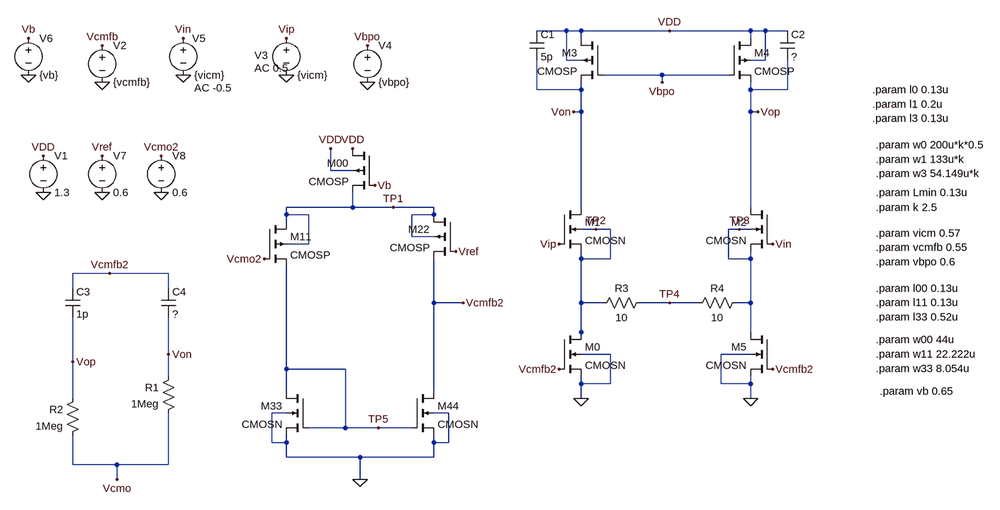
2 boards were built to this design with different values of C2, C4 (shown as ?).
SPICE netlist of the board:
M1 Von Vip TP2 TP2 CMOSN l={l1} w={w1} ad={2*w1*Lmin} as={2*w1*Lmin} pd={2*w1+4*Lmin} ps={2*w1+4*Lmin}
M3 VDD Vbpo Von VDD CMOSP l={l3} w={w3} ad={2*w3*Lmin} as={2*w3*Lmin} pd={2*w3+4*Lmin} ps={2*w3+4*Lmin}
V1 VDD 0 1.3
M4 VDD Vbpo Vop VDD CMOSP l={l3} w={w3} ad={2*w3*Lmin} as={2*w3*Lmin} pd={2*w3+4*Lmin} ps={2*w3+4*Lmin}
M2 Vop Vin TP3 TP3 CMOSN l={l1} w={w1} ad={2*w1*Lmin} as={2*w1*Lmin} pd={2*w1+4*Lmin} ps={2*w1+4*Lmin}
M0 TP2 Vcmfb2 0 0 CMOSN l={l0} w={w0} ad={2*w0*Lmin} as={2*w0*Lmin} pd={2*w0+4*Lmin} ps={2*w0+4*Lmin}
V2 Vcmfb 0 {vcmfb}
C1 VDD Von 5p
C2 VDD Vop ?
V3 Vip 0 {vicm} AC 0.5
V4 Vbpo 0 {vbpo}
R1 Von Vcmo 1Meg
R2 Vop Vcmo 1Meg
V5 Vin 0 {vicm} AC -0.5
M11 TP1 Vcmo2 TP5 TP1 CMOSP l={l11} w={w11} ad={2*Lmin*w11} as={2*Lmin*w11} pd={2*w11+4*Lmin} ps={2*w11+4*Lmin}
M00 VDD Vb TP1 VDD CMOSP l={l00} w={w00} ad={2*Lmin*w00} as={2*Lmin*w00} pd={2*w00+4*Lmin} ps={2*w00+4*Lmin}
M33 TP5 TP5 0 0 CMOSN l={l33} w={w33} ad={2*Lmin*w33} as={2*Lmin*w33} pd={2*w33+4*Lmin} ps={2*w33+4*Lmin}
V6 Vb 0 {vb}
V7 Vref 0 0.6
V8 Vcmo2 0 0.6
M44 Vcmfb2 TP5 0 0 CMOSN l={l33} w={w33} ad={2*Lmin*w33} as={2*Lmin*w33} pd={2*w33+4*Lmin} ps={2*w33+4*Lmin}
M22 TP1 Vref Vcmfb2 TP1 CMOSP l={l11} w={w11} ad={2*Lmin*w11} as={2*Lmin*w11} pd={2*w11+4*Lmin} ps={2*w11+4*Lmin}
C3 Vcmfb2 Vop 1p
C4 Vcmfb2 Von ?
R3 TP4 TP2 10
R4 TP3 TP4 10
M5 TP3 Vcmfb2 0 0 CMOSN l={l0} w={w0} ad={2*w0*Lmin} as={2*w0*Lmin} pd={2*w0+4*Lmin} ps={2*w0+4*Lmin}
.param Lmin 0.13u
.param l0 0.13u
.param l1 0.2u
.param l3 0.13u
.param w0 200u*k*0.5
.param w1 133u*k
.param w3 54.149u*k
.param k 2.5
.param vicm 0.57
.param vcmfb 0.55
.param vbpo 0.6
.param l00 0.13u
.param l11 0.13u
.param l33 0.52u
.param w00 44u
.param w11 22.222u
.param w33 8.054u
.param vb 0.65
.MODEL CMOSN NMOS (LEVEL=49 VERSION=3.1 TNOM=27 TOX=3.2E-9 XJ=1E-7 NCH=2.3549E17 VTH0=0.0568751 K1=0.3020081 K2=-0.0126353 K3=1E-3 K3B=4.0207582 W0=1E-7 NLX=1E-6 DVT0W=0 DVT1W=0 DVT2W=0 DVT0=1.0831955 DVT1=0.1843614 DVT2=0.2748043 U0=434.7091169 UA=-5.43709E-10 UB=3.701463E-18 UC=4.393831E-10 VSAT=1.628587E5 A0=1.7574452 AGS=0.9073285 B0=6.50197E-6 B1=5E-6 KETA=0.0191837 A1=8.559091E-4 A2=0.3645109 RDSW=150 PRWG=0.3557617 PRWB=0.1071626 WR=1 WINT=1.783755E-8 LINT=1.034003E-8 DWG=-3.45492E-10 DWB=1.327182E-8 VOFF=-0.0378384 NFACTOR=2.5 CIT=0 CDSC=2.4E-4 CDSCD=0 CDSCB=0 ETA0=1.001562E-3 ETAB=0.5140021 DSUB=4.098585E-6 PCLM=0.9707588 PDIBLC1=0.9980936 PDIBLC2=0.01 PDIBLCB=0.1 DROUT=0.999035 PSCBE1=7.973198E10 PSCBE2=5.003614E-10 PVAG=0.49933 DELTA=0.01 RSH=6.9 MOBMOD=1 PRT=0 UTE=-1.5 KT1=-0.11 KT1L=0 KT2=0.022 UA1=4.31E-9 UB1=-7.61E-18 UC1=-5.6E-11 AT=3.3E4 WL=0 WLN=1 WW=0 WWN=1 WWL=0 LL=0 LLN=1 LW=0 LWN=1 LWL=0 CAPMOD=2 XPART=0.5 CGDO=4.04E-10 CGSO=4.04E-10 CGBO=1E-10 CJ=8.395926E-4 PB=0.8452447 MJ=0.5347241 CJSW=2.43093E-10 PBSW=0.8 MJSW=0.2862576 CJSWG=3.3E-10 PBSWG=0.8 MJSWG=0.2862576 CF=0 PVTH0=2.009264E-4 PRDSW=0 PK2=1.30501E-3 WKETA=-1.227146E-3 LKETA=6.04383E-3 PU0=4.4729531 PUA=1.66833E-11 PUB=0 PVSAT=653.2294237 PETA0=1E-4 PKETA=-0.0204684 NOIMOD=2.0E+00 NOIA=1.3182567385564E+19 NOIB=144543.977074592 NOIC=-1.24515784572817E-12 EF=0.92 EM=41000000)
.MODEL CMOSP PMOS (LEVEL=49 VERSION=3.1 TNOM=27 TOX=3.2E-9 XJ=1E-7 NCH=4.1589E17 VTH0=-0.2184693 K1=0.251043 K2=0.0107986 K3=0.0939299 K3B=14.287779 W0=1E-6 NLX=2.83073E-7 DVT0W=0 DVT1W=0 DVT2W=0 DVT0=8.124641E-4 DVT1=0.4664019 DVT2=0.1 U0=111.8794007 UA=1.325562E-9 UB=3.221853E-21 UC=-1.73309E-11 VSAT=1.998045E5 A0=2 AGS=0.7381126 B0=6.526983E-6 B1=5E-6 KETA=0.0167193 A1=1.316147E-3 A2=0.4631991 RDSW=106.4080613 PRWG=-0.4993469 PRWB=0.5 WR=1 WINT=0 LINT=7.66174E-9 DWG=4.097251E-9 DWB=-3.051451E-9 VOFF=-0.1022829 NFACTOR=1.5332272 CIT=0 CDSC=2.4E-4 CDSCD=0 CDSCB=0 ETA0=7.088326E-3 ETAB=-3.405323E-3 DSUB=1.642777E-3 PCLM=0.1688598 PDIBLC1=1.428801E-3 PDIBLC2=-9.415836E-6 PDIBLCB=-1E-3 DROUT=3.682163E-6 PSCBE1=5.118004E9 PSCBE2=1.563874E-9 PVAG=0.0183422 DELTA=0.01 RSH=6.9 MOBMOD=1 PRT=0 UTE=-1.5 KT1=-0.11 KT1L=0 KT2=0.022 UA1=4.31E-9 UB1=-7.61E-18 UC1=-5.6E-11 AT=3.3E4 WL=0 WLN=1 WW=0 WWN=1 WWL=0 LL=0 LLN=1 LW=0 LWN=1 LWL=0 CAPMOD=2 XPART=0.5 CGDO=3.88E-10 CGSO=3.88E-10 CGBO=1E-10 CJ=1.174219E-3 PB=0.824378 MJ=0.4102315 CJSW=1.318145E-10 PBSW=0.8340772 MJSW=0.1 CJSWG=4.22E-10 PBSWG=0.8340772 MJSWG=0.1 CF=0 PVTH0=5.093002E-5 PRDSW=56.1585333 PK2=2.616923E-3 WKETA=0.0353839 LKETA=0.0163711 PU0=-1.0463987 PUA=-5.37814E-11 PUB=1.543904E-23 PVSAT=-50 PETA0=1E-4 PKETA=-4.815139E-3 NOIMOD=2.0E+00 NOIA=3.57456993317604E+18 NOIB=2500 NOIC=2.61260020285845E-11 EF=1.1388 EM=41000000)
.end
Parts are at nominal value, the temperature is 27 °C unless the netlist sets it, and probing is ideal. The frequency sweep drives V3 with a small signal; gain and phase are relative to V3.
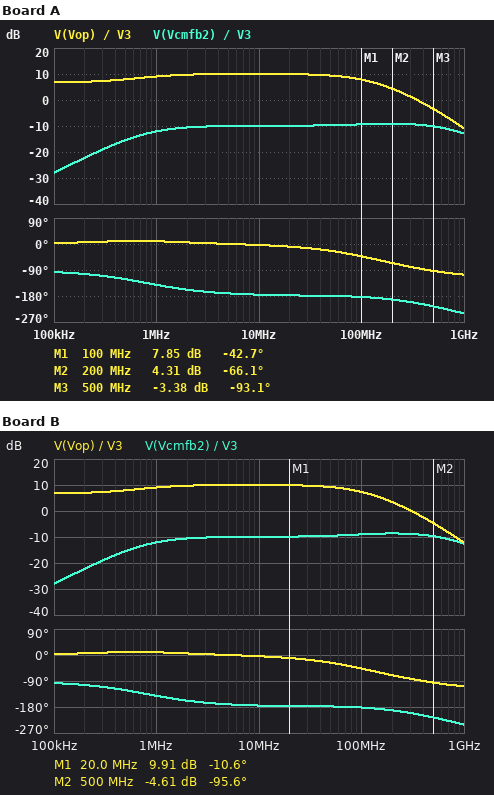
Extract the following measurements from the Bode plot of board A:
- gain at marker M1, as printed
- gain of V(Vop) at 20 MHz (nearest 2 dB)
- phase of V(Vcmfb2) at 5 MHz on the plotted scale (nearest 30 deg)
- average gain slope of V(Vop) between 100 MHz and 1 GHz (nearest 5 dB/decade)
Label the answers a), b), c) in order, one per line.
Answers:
a) 7.85 dB
b) 10 dB
c) -180 deg
d) -20 dB/decade
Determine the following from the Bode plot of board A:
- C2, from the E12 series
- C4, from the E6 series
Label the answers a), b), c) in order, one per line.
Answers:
a) 10 pF
b) 3.3 pF
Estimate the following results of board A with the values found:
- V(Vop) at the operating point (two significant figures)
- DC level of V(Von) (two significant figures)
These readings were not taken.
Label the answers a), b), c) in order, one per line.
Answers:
a) 1.1 V
b) 1.1 V
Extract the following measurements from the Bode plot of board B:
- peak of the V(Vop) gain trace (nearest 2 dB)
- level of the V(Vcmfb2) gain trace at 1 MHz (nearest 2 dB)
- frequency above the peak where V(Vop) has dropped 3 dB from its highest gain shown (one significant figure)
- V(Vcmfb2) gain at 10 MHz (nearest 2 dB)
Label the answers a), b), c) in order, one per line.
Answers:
a) 10 dB
b) -12 dB
c) 100 MHz
d) -10 dB
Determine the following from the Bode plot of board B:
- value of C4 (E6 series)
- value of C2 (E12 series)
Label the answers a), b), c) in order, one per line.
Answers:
a) 3.3 pF
b) 12 pF
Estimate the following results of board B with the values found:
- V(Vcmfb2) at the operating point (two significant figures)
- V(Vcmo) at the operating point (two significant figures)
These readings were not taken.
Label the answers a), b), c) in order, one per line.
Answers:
a) 550 mV
b) 1.1 V
